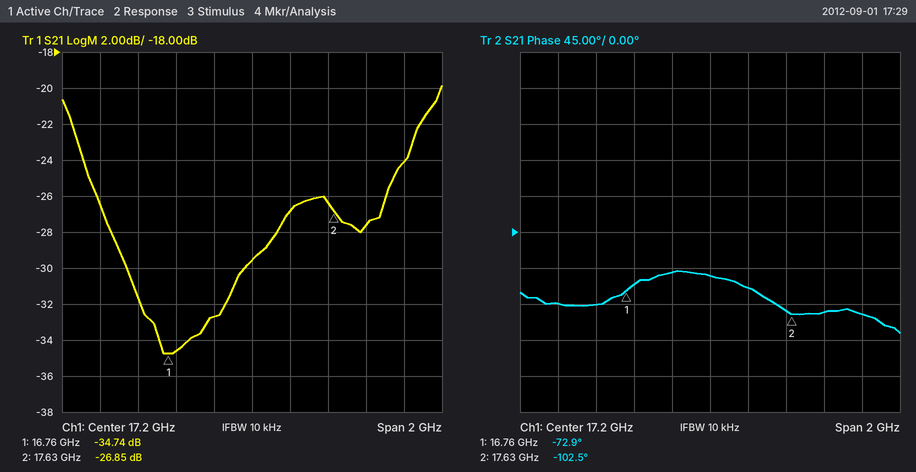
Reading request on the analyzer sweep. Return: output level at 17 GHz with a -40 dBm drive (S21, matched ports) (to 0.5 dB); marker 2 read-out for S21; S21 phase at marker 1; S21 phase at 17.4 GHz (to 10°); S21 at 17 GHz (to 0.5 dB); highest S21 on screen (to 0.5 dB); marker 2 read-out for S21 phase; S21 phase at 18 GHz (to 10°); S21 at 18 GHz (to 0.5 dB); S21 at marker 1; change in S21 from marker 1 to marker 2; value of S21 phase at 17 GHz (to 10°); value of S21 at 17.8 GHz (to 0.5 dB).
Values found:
-72.5 dBm
-26.85 dB
-72.9°
-70°
-32.5 dB
-20.0 dB
-102.5°
-100°
-24.0 dB
-34.74 dB
7.89 dB
-50°
-27.5 dB
